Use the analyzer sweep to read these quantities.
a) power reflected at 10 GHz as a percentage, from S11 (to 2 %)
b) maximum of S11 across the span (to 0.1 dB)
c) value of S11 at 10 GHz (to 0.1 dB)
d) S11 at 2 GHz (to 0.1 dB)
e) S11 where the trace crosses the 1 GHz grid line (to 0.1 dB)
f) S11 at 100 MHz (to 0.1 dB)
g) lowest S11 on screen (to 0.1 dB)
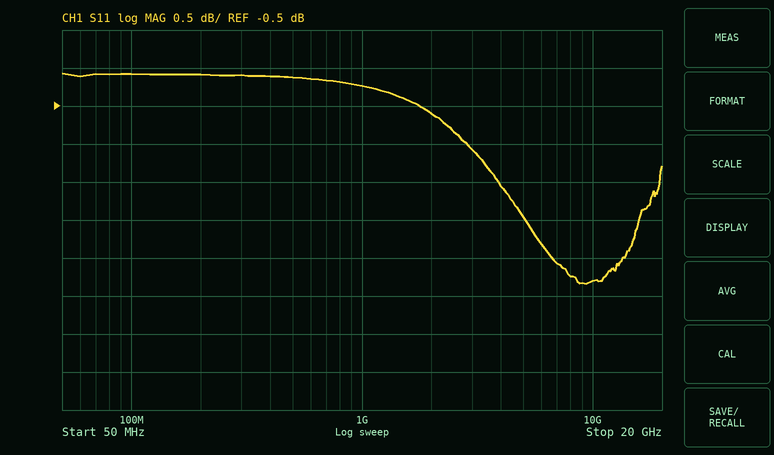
52 %
-0.1 dB
-2.8 dB
-0.6 dB
-0.2 dB
-0.1 dB
-2.8 dB
